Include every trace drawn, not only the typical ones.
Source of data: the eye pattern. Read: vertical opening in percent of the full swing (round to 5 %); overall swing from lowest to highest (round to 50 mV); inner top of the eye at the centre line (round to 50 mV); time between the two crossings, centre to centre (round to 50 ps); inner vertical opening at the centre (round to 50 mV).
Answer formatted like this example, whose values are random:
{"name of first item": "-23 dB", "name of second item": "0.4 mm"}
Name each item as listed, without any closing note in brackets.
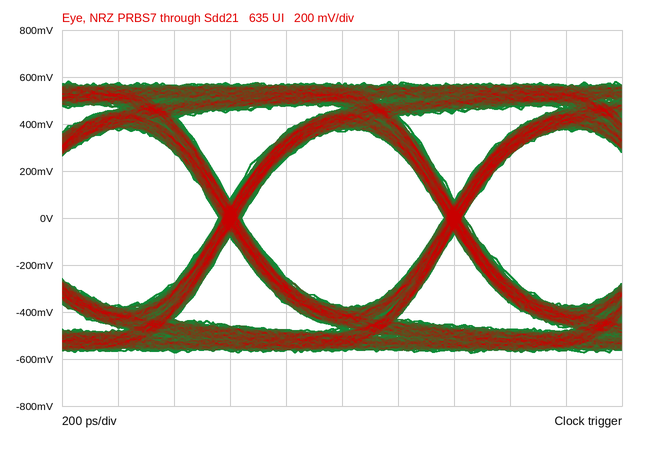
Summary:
{"vertical opening in percent of the full swing": "65 %", "overall swing from lowest to highest": "1.15 V", "inner top of the eye at the centre line": "350 mV", "time between the two crossings, centre to centre": "800 ps", "inner vertical opening at the centre": "750 mV"}
